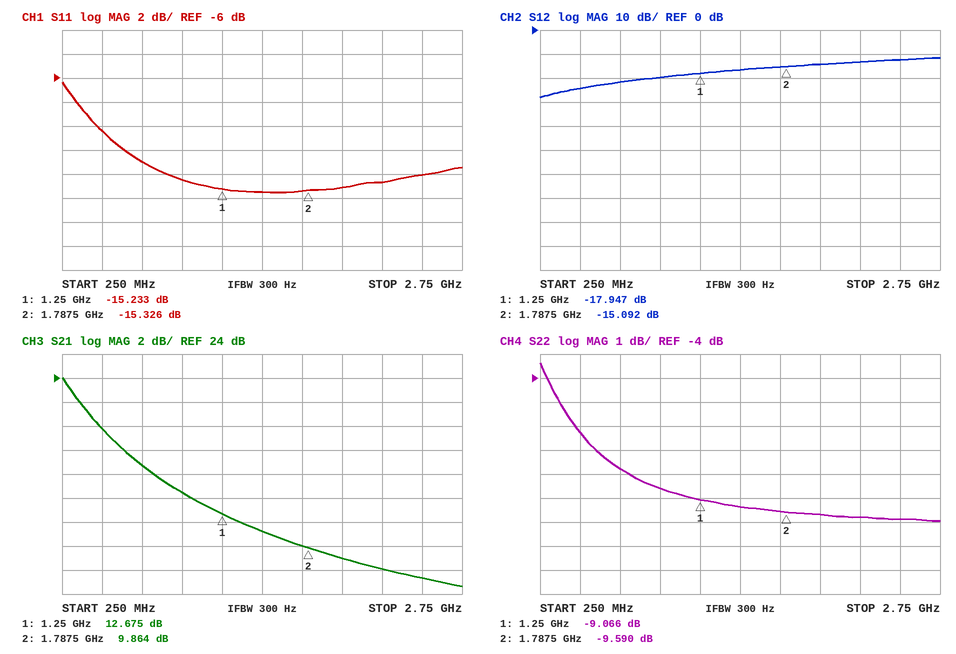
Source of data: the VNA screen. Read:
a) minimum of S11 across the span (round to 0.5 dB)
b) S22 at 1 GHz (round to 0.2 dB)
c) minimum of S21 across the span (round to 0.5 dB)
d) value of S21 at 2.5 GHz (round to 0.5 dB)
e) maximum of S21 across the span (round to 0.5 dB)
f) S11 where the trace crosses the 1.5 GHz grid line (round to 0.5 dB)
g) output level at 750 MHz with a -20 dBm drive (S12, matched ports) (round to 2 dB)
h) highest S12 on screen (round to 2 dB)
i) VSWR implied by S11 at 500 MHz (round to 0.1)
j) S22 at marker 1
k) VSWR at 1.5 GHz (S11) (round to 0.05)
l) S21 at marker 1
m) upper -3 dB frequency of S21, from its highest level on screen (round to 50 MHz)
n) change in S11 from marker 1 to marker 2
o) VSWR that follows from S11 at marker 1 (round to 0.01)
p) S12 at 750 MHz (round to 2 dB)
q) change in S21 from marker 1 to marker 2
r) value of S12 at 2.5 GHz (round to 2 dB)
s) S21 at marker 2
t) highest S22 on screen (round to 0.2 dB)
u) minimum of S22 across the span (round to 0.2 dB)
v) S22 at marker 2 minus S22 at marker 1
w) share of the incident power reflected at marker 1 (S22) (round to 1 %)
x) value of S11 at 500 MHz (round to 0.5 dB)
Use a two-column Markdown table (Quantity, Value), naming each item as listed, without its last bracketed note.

| Quantity | Value |
|---|---|
| minimum of S11 across the span | -15.5 dB |
| S22 at 1 GHz | -8.6 dB |
| minimum of S21 across the span | 6.5 dB |
| value of S21 at 2.5 GHz | 7.5 dB |
| maximum of S21 across the span | 24.0 dB |
| S11 where the trace crosses the 1.5 GHz grid line | -15.5 dB |
| output level at 750 MHz with a -20 dBm drive (S12, matched ports) | -42 dBm |
| highest S12 on screen | -12 dB |
| VSWR implied by S11 at 500 MHz | 1.9 |
| S22 at marker 1 | -9.066 dB |
| VSWR at 1.5 GHz (S11) | 1.40 |
| S21 at marker 1 | 12.675 dB |
| upper -3 dB frequency of S21, from its highest level on screen | 400 MHz |
| change in S11 from marker 1 to marker 2 | -0.093 dB |
| VSWR that follows from S11 at marker 1 | 1.42 |
| S12 at 750 MHz | -22 dB |
| change in S21 from marker 1 to marker 2 | -2.811 dB |
| value of S12 at 2.5 GHz | -12 dB |
| S21 at marker 2 | 9.864 dB |
| highest S22 on screen | -3.4 dB |
| minimum of S22 across the span | -10.0 dB |
| S22 at marker 2 minus S22 at marker 1 | -0.524 dB |
| share of the incident power reflected at marker 1 (S22) | 12 % |
| value of S11 at 500 MHz | -10.5 dB |
